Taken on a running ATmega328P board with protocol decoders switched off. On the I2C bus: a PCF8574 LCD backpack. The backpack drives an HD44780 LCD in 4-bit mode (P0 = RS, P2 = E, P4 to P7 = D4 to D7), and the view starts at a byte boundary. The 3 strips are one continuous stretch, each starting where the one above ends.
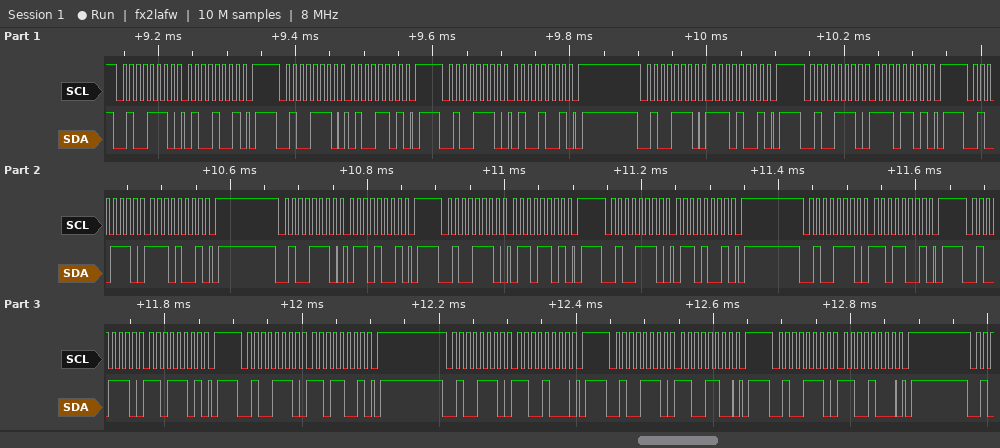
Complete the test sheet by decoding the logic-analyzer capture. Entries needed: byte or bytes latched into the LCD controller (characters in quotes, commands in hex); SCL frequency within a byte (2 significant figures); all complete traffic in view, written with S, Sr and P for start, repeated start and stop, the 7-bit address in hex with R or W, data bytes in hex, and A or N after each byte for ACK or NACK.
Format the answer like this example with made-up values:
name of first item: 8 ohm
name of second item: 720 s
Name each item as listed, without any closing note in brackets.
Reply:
byte or bytes latched into the LCD controller: 'N' 'm'
SCL frequency within a byte: 100 kHz
all complete traffic in view, written with S, Sr and P for start, repeated start and stop, the 7-bit address in hex with R or W, data bytes in hex, and A or N after each byte for ACK or NACK: S 27W A 49 A P S 27W A 4D A P S 27W A 49 A P S 27W A E9 A P S 27W A ED A P S 27W A E9 A P S 27W A 69 A P S 27W A 6D A P S 27W A 69 A P S 27W A D9 A P S 27W A DD A P S 27W A D9 A P S 27W A C8 A P S 27W A CC A P S 27W A C8 A P
